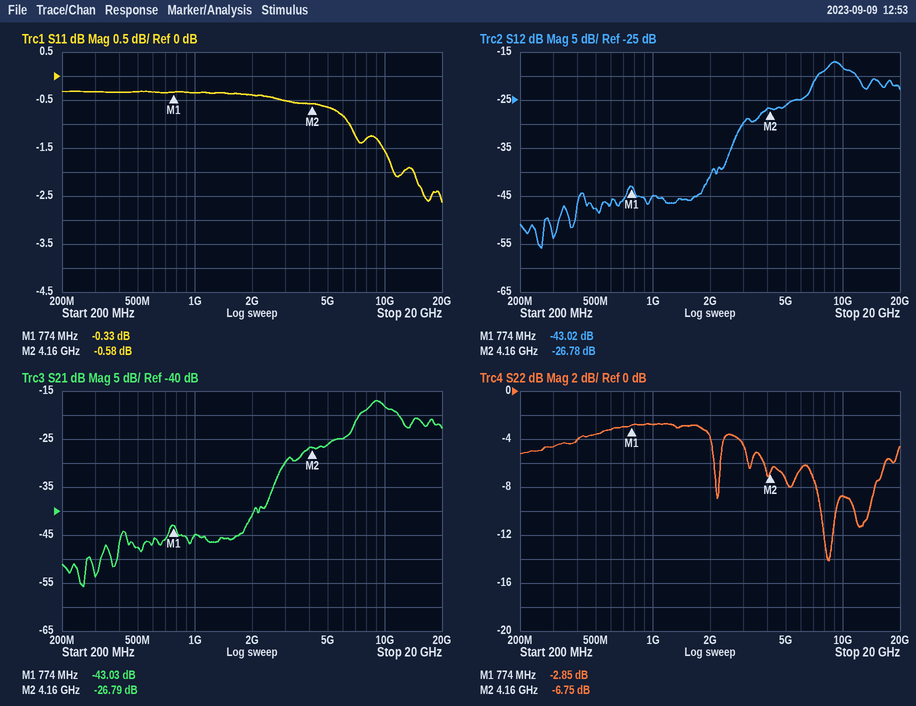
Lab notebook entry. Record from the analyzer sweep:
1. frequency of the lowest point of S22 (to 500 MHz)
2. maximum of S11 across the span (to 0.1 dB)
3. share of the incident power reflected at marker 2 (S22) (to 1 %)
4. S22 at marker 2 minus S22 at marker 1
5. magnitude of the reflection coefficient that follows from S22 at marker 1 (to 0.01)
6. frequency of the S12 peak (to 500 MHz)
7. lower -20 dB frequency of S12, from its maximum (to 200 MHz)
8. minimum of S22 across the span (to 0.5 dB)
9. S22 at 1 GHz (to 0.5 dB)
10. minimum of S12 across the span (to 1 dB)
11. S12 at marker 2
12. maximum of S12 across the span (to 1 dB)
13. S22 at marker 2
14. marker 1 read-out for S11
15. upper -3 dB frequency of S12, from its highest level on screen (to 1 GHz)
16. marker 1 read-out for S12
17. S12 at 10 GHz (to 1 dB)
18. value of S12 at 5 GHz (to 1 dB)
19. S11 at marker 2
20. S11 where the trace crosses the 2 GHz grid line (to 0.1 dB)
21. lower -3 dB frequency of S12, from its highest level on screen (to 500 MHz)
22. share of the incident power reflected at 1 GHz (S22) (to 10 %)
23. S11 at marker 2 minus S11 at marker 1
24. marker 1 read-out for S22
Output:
8.5 GHz
-0.3 dB
21 %
-3.90 dB
0.72
9.0 GHz
2.4 GHz
-14.0 dB
-3.0 dB
-56 dB
-26.78 dB
-17 dB
-6.75 dB
-0.33 dB
12 GHz
-43.02 dB
-18 dB
-26 dB
-0.58 dB
-0.4 dB
7.5 GHz
50 %
-0.25 dB
-2.85 dB
